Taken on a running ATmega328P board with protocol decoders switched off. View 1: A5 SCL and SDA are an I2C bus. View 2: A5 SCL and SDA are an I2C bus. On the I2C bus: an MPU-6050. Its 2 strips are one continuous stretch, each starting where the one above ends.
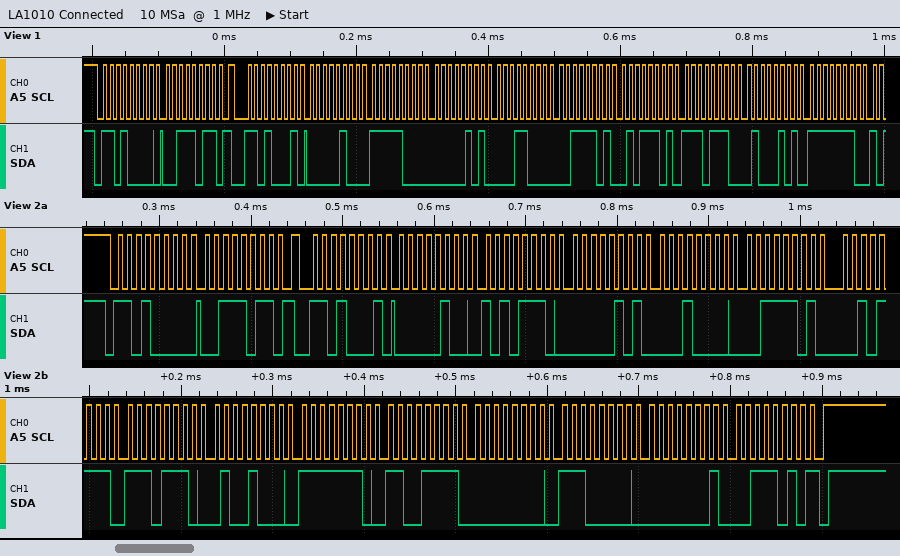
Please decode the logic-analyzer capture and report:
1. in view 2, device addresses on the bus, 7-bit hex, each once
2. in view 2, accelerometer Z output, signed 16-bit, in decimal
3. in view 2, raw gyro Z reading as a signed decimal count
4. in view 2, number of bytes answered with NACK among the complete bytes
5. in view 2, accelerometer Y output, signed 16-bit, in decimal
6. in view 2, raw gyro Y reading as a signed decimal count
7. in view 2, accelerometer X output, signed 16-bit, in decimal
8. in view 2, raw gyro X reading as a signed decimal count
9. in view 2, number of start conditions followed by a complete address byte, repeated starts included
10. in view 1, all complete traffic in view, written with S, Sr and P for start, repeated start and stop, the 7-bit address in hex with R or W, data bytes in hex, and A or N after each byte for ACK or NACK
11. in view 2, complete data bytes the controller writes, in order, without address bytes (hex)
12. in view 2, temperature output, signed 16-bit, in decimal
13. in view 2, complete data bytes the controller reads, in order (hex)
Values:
0x68
15663
314
1
1296
224
1198
-305
2
S 68W A 3B A Sr 68R A 04 A F8 A 05 A 18 A 3D A 5D A EE A 45 A FE A
3B
-4536
04 AE 05 10 3D 2F EE 48 FE CF 00 E0 01 3A
